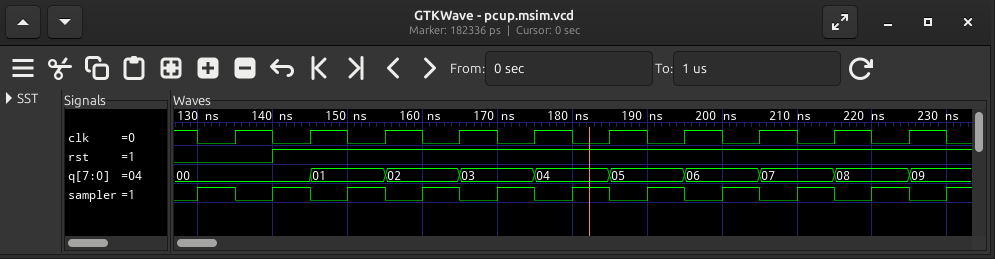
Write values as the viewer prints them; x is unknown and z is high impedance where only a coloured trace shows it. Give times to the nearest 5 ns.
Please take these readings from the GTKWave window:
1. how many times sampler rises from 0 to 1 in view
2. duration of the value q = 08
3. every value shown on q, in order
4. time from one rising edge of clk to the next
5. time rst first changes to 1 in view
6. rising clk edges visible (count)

11
10 ns
00, 01, 02, 03, 04, 05, 06, 07, 08, 09
10 ns
140 ns
10
